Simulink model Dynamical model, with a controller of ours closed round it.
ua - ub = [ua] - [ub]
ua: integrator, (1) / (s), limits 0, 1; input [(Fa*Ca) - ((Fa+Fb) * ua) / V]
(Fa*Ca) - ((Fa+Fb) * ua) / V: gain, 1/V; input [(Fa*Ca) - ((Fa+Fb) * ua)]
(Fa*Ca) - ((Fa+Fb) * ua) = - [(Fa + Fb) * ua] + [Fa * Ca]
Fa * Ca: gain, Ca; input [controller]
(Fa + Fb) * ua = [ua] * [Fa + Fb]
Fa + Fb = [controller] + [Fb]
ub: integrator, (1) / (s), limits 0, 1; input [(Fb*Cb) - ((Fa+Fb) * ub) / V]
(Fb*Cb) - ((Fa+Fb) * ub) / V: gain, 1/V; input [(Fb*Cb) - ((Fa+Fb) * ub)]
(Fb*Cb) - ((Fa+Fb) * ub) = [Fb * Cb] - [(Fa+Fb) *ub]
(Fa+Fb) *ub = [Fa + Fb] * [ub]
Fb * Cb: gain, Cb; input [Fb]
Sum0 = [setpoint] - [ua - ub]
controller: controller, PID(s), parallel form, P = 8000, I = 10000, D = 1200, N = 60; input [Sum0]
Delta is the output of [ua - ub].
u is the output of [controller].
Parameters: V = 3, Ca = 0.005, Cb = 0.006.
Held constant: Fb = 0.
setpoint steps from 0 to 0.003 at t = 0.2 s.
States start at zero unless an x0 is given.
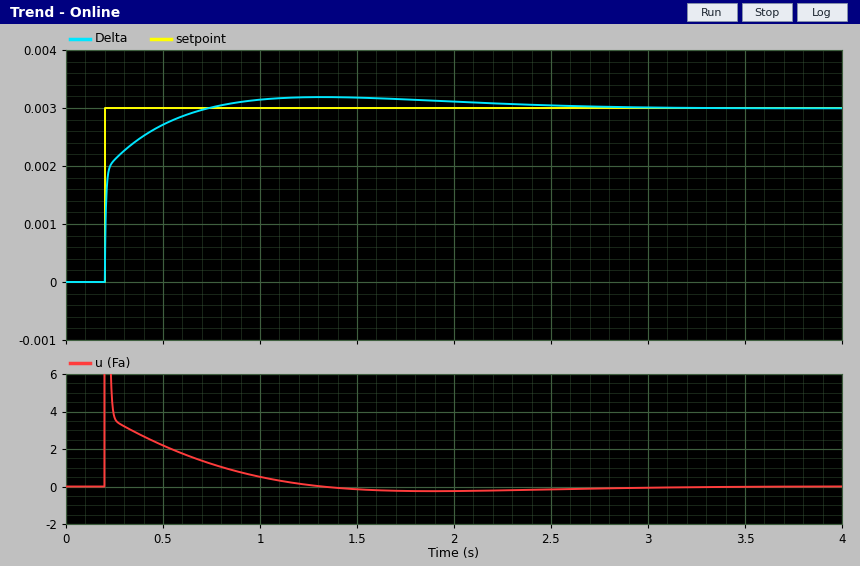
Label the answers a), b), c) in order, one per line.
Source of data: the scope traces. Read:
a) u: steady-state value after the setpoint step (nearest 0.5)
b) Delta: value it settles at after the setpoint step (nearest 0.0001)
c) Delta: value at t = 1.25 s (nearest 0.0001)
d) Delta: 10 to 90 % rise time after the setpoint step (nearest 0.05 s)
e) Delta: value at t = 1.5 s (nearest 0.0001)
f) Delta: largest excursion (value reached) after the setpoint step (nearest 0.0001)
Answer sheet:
a) 0.0
b) 0.0030
c) 0.0032
d) 0.30 s
e) 0.0032
f) 0.0032
